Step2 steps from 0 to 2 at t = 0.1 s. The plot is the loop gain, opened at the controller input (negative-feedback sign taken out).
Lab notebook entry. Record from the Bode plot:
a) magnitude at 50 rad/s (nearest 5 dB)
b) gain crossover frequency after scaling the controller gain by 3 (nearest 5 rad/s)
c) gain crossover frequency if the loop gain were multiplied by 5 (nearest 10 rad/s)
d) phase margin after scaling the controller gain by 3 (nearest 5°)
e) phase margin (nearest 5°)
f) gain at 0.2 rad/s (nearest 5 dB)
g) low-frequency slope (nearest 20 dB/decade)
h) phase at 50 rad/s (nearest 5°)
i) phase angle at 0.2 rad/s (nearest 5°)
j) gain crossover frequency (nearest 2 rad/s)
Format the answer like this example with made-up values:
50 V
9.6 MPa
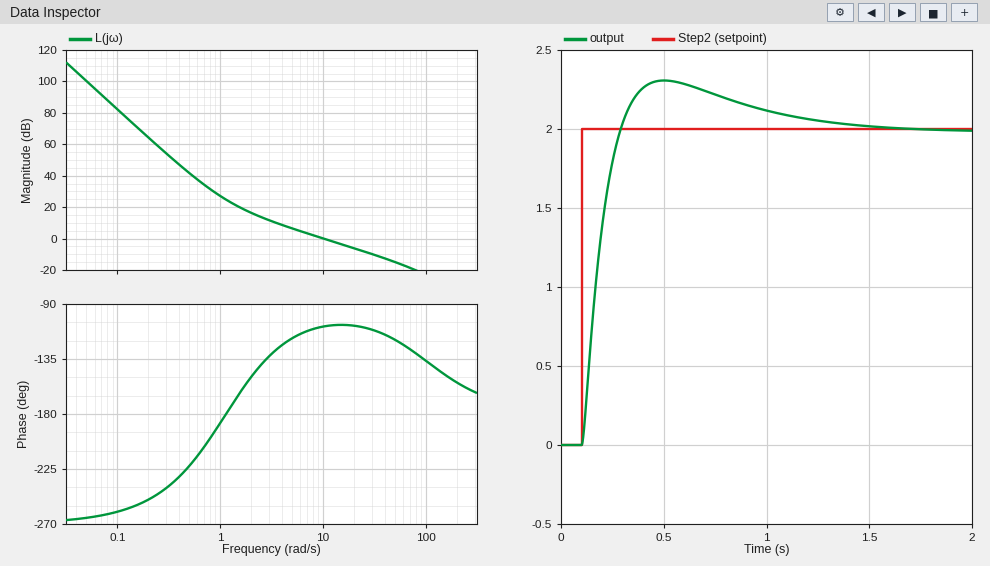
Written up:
-15 dB
30 rad/s
50 rad/s
70°
70°
65 dB
-60 dB/decade
-120°
-250°
10 rad/s
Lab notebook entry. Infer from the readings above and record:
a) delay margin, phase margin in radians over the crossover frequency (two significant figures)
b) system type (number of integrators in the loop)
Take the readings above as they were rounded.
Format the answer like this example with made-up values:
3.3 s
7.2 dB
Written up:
0.12 s
3
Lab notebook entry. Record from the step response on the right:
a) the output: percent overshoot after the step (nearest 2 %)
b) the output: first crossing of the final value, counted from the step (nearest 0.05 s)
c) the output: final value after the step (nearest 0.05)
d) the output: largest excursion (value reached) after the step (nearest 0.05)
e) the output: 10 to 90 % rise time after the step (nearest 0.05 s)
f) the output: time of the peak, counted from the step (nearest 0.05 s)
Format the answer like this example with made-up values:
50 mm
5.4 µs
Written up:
16 %
0.20 s
2.00
2.30
0.15 s
0.40 s
